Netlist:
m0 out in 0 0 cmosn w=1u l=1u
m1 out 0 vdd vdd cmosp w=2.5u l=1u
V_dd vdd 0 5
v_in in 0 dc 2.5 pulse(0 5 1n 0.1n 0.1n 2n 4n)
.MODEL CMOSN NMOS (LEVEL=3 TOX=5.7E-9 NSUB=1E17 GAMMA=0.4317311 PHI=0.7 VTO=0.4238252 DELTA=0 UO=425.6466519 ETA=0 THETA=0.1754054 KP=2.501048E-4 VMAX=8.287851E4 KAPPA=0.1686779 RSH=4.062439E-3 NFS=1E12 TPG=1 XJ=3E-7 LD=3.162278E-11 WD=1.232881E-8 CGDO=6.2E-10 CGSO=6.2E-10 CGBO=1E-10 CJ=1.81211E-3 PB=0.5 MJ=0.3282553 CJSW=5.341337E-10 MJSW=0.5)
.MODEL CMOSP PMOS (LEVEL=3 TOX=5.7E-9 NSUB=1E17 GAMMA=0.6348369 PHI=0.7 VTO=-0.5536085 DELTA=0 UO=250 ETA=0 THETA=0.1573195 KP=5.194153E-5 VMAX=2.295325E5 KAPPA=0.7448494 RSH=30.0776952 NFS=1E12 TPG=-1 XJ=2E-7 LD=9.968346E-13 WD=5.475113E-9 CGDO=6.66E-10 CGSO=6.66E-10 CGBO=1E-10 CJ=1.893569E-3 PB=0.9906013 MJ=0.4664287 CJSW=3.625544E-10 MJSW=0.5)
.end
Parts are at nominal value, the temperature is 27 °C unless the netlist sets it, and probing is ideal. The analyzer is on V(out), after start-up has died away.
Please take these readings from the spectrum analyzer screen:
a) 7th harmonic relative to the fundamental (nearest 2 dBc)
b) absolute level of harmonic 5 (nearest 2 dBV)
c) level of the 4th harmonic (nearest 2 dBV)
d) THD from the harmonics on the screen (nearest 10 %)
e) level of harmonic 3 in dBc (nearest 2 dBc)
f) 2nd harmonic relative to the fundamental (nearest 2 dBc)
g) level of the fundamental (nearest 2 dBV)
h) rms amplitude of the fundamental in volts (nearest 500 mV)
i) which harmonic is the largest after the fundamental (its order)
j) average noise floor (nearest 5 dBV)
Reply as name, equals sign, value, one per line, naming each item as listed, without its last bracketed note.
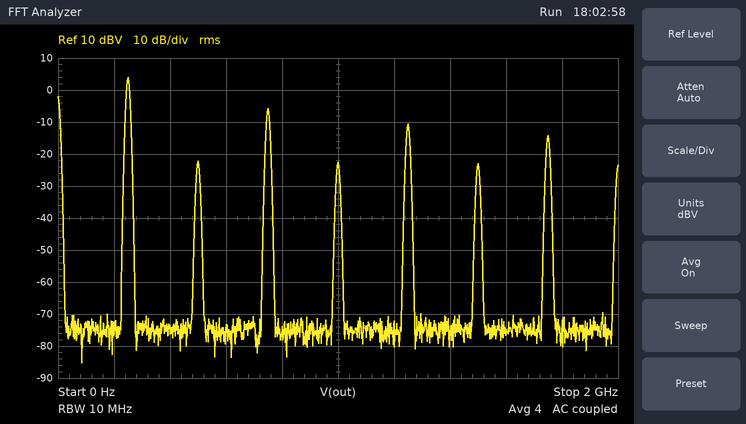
7th harmonic relative to the fundamental = -18 dBc
absolute level of harmonic 5 = -10 dBV
level of the 4th harmonic = -22 dBV
THD from the harmonics on the screen = 40 %
level of harmonic 3 in dBc = -10 dBc
2nd harmonic relative to the fundamental = -26 dBc
level of the fundamental = 4 dBV
rms amplitude of the fundamental in volts = 1.5 V
which harmonic is the largest after the fundamental = 3
average noise floor = -75 dBV
